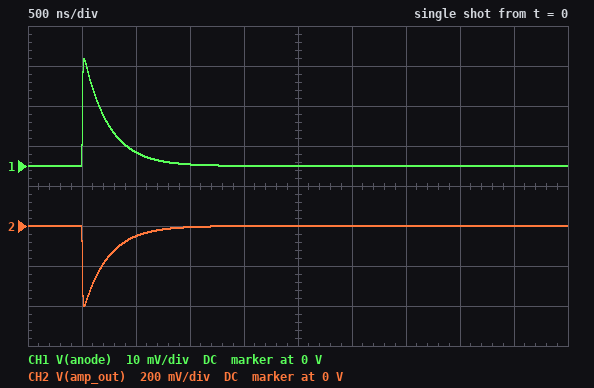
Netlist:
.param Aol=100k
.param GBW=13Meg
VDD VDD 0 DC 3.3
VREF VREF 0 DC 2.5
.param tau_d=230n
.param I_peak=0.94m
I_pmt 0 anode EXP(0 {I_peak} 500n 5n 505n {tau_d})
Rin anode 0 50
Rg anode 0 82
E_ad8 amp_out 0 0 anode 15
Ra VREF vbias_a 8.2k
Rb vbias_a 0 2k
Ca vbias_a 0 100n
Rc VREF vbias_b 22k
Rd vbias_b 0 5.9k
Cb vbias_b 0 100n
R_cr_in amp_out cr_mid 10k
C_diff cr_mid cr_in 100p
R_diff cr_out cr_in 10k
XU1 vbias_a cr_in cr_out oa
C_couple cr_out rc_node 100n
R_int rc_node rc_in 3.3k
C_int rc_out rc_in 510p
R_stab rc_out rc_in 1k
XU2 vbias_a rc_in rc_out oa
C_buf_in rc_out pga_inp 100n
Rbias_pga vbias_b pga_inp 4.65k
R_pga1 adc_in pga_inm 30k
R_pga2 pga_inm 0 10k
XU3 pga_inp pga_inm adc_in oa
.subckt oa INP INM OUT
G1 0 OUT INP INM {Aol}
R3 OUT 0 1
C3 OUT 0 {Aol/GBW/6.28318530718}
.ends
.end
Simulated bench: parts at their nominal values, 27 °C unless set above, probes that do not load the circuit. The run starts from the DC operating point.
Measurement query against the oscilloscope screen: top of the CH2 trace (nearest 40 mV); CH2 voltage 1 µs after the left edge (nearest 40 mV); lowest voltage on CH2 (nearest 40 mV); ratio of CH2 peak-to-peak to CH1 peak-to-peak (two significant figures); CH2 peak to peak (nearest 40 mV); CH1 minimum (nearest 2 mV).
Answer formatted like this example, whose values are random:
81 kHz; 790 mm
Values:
0 V; -40 mV; -400 mV; 15; 400 mV; 0 V
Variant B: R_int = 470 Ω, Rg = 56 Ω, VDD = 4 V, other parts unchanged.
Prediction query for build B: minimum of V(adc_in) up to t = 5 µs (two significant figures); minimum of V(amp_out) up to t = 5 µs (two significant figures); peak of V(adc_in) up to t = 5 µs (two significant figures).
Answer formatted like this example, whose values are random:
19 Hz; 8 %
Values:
1.5 V; -340 mV; 2.3 V
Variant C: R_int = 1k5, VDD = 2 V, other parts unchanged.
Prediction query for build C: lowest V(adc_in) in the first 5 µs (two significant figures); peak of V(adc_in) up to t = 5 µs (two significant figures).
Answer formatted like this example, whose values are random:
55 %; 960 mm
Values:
1.9 V; 2.2 V
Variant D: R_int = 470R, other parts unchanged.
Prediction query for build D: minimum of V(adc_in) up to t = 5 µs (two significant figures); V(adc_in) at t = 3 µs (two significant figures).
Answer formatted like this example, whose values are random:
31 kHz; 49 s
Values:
1.4 V; 2.3 V
